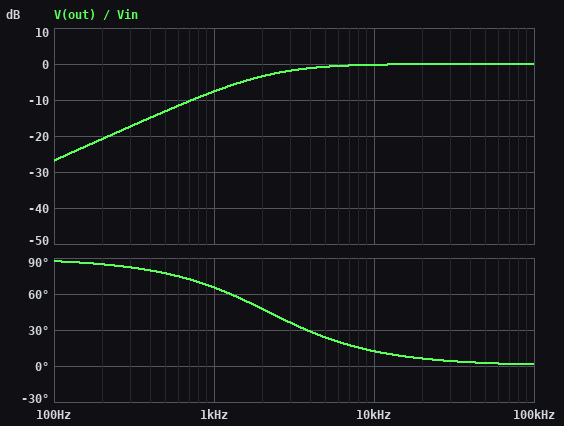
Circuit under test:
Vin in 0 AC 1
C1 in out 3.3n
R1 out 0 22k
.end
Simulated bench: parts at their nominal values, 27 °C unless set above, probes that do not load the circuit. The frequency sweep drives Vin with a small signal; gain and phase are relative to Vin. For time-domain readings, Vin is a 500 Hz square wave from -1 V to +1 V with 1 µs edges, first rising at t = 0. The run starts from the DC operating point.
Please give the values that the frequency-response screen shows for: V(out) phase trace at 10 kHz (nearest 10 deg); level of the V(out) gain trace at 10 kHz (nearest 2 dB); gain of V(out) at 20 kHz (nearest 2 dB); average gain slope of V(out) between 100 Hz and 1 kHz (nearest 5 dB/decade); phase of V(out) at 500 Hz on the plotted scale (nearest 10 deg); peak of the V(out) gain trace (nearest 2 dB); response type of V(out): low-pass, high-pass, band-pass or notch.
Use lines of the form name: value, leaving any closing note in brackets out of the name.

V(out) phase trace at 10 kHz: 10 deg
level of the V(out) gain trace at 10 kHz: 0 dB
gain of V(out) at 20 kHz: 0 dB
average gain slope of V(out) between 100 Hz and 1 kHz: 20 dB/decade
phase of V(out) at 500 Hz on the plotted scale: 80 deg
peak of the V(out) gain trace: 0 dB
response type of V(out): low-pass, high-pass, band-pass or notch: high-pass
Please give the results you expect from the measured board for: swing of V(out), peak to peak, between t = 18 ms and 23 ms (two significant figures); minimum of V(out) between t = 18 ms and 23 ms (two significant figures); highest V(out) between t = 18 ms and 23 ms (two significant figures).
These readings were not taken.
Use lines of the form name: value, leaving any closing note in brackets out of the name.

swing of V(out), peak to peak, between t = 18 ms and 23 ms: 4.0 V
minimum of V(out) between t = 18 ms and 23 ms: -2.0 V
highest V(out) between t = 18 ms and 23 ms: 2.0 V
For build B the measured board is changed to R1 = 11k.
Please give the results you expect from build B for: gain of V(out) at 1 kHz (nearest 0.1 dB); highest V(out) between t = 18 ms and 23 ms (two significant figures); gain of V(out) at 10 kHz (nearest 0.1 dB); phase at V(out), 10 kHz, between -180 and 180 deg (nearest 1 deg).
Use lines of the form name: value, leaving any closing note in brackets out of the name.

gain of V(out) at 1 kHz: -13.1 dB
highest V(out) between t = 18 ms and 23 ms: 2.0 V
gain of V(out) at 10 kHz: -0.8 dB
phase at V(out), 10 kHz, between -180 and 180 deg: 24 deg
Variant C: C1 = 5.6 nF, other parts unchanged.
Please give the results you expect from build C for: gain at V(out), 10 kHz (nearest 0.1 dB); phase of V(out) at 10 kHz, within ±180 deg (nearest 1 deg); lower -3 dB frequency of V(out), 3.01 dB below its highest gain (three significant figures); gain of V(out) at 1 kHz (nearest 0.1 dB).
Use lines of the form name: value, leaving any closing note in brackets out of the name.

gain at V(out), 10 kHz: -0.1 dB
phase of V(out) at 10 kHz, within ±180 deg: 7 deg
lower -3 dB frequency of V(out), 3.01 dB below its highest gain: 1.29 kHz
gain of V(out) at 1 kHz: -4.3 dB
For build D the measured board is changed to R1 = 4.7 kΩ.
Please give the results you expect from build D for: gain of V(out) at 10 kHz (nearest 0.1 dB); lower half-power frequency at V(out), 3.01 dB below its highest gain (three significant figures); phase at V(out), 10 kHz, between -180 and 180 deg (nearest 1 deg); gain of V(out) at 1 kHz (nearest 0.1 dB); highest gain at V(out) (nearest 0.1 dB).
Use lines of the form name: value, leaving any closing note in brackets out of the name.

gain of V(out) at 10 kHz: -3.1 dB
lower half-power frequency at V(out), 3.01 dB below its highest gain: 10.3 kHz
phase at V(out), 10 kHz, between -180 and 180 deg: 46 deg
gain of V(out) at 1 kHz: -20.3 dB
highest gain at V(out): 0 dB
